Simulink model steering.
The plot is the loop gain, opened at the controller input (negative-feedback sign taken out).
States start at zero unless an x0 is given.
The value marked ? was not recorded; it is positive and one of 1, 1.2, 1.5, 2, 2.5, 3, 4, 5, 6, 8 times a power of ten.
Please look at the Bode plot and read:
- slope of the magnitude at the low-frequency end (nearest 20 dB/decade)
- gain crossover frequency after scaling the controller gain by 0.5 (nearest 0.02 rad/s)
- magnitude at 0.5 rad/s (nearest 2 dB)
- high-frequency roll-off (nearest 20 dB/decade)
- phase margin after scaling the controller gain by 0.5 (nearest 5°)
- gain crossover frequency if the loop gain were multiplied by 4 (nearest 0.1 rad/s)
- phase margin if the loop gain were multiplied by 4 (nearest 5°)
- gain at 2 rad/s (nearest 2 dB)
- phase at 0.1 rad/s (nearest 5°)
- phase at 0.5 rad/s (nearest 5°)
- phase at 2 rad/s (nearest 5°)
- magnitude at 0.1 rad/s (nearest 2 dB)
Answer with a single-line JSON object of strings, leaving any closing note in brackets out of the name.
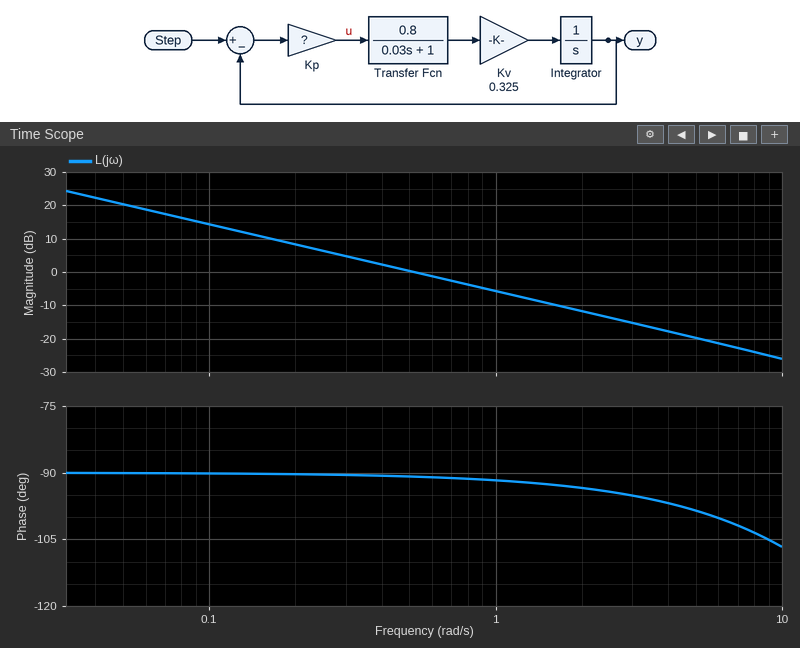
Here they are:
{"slope of the magnitude at the low-frequency end": "-20 dB/decade", "gain crossover frequency after scaling the controller gain by 0.5": "0.26 rad/s", "magnitude at 0.5 rad/s": "0 dB", "high-frequency roll-off": "-20 dB/decade", "phase margin after scaling the controller gain by 0.5": "90°", "gain crossover frequency if the loop gain were multiplied by 4": "2.1 rad/s", "phase margin if the loop gain were multiplied by 4": "85°", "gain at 2 rad/s": "-12 dB", "phase at 0.1 rad/s": "-90°", "phase at 0.5 rad/s": "-90°", "phase at 2 rad/s": "-95°", "magnitude at 0.1 rad/s": "14 dB"}
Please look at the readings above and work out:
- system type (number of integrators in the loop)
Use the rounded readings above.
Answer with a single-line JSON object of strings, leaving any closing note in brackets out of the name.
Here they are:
{"system type": "1"}
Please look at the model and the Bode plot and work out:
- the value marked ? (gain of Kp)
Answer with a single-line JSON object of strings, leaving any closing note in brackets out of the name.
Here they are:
{"the value marked ?": "2"}
